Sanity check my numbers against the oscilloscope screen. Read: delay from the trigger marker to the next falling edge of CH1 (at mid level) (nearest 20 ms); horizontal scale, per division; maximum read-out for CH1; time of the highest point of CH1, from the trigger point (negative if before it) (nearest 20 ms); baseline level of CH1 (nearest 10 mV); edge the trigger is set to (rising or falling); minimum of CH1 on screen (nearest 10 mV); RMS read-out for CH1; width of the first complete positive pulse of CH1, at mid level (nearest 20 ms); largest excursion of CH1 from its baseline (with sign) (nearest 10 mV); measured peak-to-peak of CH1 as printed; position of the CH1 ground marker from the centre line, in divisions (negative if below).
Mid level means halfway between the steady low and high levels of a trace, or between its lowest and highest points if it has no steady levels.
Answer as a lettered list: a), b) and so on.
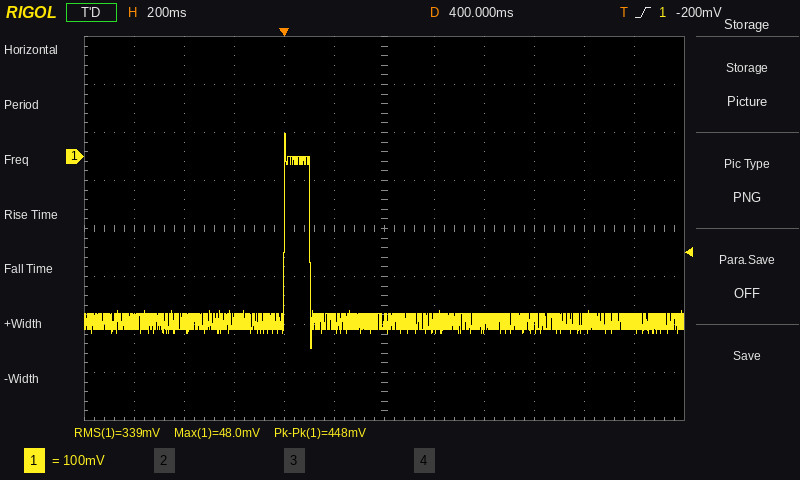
a) 100 ms
b) 200 ms
c) 48.0 mV
d) 0 ms
e) -340 mV
f) rising
g) -400 mV
h) 339 mV
i) 100 ms
j) +390 mV
k) 448 mV
l) +1.5 div
